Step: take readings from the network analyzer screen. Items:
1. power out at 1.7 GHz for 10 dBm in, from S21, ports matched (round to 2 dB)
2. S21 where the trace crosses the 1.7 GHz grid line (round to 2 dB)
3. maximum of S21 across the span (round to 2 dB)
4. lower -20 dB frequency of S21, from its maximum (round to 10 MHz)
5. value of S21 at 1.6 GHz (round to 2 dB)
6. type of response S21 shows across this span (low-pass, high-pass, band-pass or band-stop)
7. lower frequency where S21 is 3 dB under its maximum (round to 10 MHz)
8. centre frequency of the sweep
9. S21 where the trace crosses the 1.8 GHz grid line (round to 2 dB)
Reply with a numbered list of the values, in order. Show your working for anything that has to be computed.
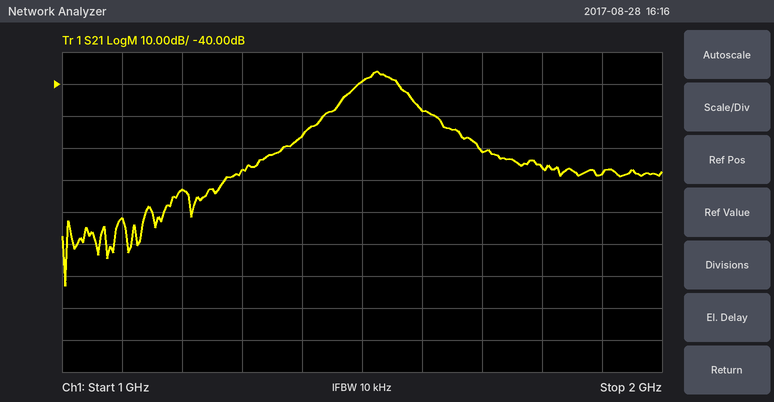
1. 10 dBm + (-62 dB) = -52 dBm
2. -62 dB
3. -36 dB
4. 1.40 GHz
5. -48 dB
6. band-pass
7. 1.50 GHz
8. 1.5 GHz
9. -66 dB
